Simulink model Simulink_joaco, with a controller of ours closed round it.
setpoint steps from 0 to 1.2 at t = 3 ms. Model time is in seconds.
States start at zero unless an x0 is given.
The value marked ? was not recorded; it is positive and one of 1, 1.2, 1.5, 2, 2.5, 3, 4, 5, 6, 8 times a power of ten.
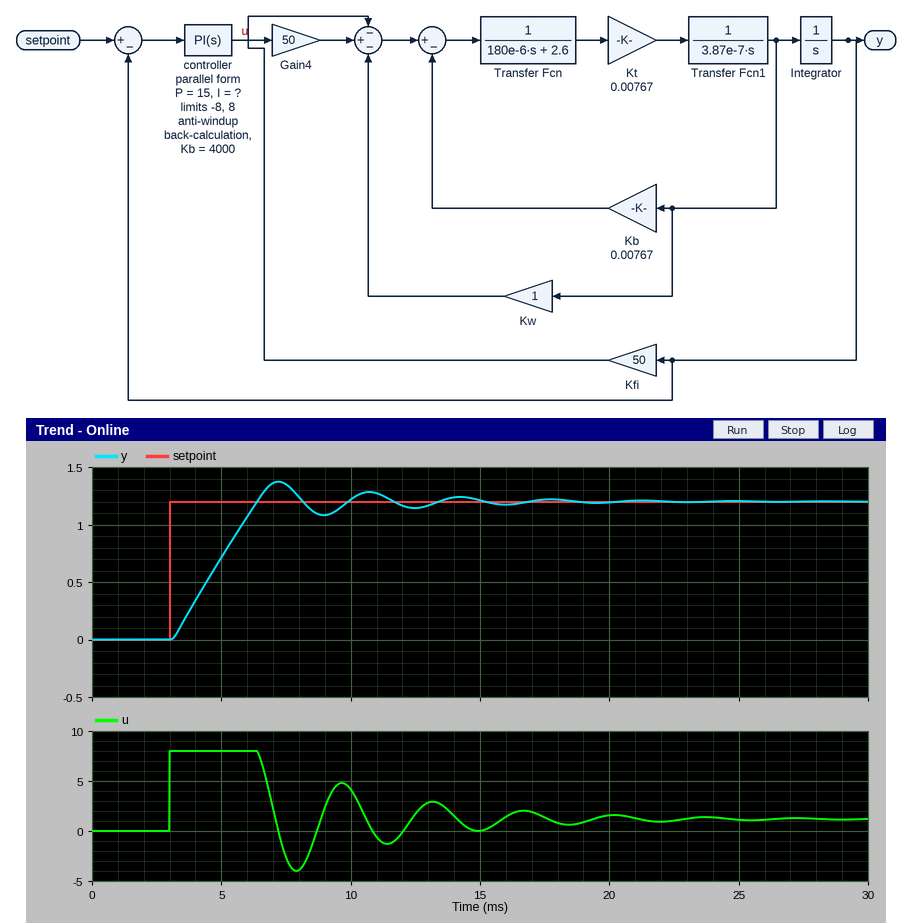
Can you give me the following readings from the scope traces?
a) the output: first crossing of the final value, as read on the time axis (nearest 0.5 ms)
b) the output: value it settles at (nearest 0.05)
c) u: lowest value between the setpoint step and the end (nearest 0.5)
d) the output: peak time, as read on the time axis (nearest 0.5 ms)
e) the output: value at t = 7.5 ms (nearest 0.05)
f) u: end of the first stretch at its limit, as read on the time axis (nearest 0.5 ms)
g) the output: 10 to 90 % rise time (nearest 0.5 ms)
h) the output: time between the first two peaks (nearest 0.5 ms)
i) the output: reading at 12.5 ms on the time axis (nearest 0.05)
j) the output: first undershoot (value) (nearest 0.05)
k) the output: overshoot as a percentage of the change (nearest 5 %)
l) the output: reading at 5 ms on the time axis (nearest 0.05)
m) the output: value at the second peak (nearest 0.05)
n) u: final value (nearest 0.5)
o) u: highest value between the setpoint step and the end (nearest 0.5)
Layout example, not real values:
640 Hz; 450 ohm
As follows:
6.5 ms; 1.20; -4.0; 7.0 ms; 1.35; 6.5 ms; 2.5 ms; 3.5 ms; 1.15; 1.10; 15 %; 0.70; 1.30; 1.0; 8.0
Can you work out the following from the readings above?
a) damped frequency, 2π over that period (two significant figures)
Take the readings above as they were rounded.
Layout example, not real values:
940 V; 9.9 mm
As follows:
1.8 rad/ms
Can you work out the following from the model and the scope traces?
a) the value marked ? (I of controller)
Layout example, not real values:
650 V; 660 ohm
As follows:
60000
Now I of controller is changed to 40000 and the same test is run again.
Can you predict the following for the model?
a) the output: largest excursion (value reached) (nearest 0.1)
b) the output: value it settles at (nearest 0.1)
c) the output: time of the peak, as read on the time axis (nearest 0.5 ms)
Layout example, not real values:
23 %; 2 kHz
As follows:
1.4; 1.2; 7.5 ms
